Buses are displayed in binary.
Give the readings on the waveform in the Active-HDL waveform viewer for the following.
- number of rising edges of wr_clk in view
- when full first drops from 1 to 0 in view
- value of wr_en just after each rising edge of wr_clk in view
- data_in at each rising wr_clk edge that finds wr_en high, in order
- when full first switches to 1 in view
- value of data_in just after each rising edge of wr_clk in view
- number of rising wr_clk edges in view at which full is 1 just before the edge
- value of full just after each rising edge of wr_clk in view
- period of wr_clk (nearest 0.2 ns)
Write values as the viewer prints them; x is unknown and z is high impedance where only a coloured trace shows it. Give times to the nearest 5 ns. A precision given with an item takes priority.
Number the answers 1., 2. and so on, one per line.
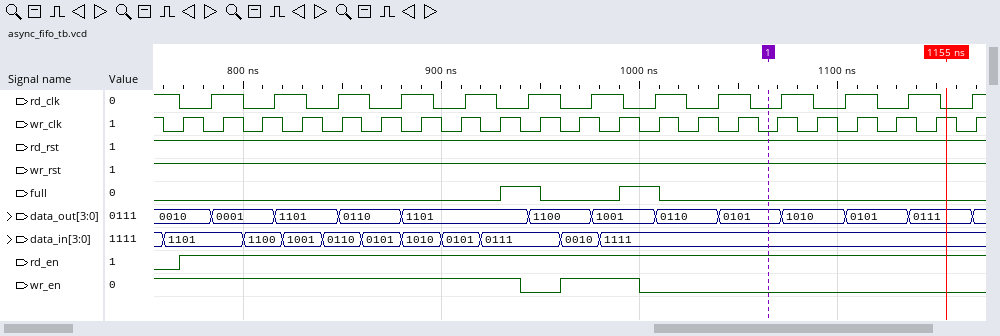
1. 21
2. 950 ns
3. 1 1 1 1 1 1 1 1 1 0 1 1 0 0 0 0 0 0 0 0 0
4. 1101, 1101, 1100, 1001, 0110, 0101, 1010, 0101, 0111, 0010, 1111
5. 930 ns
6. 1101, 1101, 1100, 1001, 0110, 0101, 1010, 0101, 0111, 0111, 0010, 1111, 1111, 1111, 1111, 1111, 1111, 1111, 1111, 1111, 1111
7. 2
8. 0 0 0 0 0 0 0 0 1 0 0 1 0 0 0 0 0 0 0 0 0
9. 20 ns
